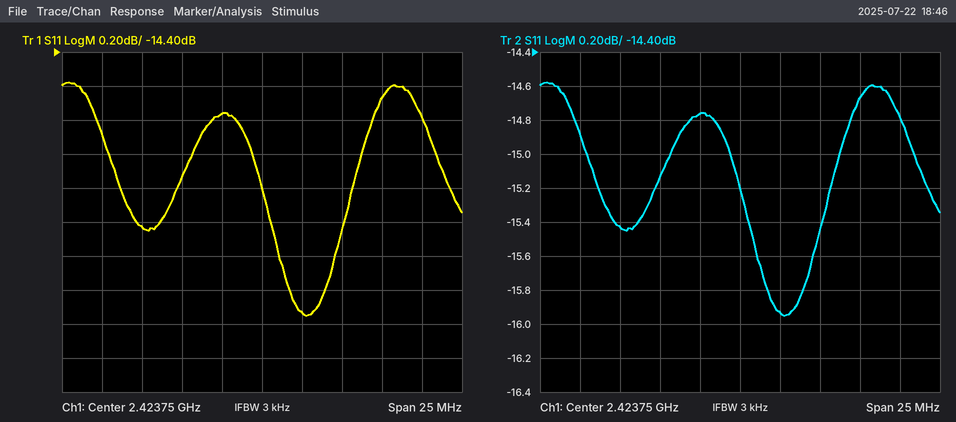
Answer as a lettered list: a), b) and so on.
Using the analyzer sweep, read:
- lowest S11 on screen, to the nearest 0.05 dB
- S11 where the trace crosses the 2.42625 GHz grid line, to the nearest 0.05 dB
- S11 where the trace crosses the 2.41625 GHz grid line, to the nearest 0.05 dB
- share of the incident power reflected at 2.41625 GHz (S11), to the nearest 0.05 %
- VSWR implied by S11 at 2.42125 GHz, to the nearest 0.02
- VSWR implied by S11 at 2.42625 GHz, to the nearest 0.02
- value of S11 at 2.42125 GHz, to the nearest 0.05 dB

a) -15.95 dB
b) -15.95 dB
c) -15.45 dB
d) 2.85 %
e) 1.44
f) 1.38
g) -14.75 dB
